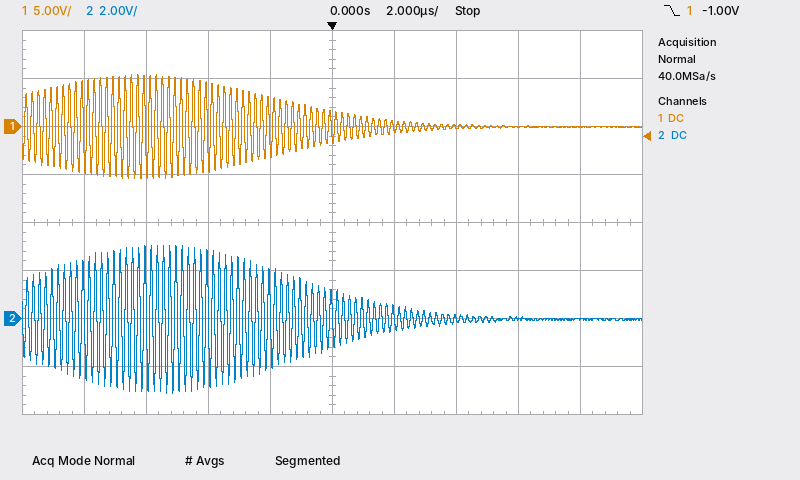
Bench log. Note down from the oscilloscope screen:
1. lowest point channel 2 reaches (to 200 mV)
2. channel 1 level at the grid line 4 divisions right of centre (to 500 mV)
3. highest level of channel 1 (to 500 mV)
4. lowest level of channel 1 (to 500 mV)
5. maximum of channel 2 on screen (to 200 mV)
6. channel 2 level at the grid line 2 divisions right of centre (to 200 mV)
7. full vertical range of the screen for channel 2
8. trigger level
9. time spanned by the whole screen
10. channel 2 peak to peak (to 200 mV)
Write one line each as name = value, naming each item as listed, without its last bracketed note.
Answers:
lowest point channel 2 reaches = -3.2 V
channel 1 level at the grid line 4 divisions right of centre = 0.0 V
highest level of channel 1 = 5.5 V
lowest level of channel 1 = -5.5 V
maximum of channel 2 on screen = 3.0 V
channel 2 level at the grid line 2 divisions right of centre = 0.0 V
full vertical range of the screen for channel 2 = 16 V
trigger level = -1.00 V
time spanned by the whole screen = 20 µs
channel 2 peak to peak = 6.2 V
